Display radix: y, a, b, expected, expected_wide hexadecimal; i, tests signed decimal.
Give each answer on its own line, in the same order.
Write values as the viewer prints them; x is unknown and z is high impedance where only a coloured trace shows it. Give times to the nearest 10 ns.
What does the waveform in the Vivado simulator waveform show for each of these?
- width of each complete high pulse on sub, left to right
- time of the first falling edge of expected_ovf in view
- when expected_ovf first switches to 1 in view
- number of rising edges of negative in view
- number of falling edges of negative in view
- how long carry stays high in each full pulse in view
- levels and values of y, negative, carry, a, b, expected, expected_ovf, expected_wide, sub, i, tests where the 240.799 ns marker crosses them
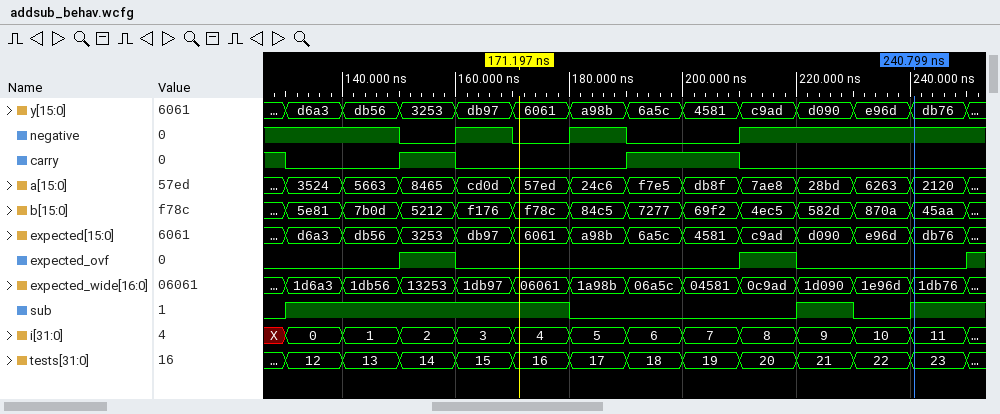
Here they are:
50 ns, 10 ns
160 ns
150 ns
3
3
10 ns, 20 ns
y=db76, negative=1, carry=0, a=2120, b=45aa, expected=db76, expected_ovf=0, expected_wide=1db76, sub=1, i=11, tests=23
